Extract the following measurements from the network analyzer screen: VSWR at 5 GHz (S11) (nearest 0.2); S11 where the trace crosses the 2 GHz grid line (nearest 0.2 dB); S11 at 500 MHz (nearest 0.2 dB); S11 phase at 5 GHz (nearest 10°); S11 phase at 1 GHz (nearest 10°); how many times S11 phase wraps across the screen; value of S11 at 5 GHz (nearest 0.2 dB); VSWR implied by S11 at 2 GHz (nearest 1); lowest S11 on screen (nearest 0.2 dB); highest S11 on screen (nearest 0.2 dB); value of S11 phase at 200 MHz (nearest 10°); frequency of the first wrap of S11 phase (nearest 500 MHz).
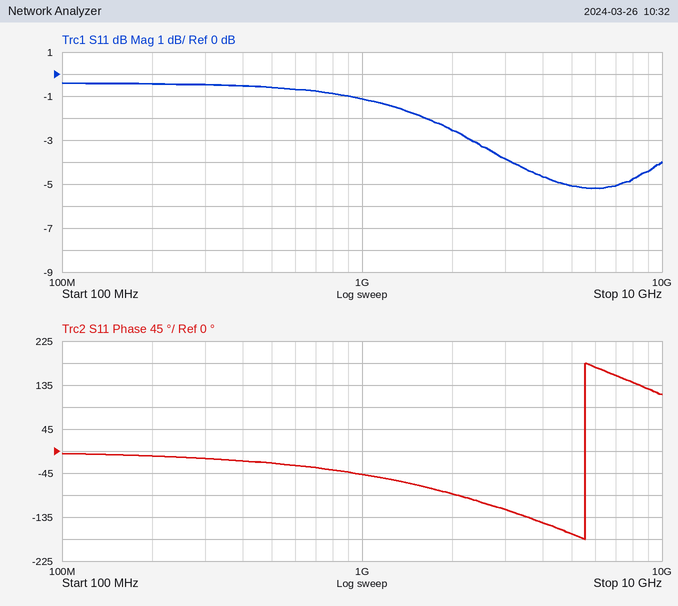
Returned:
3.6
-2.6 dB
-0.6 dB
-170°
-50°
1
-5.0 dB
7
-5.2 dB
-0.4 dB
-10°
5.5 GHz
